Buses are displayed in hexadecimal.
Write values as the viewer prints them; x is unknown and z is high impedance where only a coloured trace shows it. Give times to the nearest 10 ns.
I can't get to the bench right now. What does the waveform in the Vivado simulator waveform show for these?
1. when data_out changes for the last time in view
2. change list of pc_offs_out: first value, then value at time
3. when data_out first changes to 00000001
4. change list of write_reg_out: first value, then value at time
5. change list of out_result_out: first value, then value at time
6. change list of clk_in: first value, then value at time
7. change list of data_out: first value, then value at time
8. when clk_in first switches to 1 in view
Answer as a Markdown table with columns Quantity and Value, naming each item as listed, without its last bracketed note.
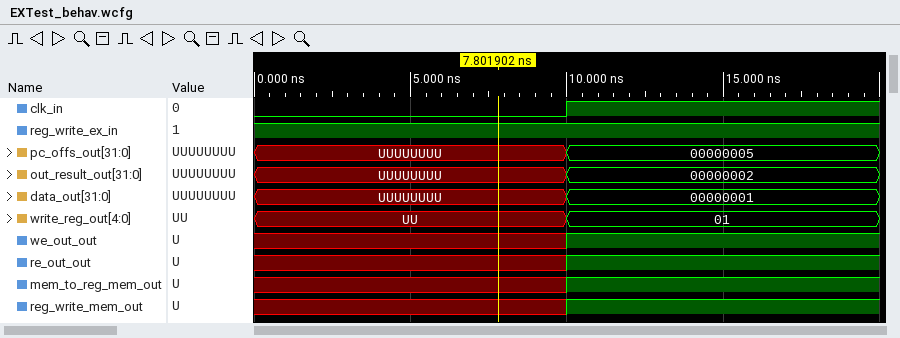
| Quantity | Value |
|---|---|
| when data_out changes for the last time in view | 10 ns |
| change list of pc_offs_out: first value, then value at time | UUUUUUUU, 00000005 at 10 ns |
| when data_out first changes to 00000001 | 10 ns |
| change list of write_reg_out: first value, then value at time | UU, 01 at 10 ns |
| change list of out_result_out: first value, then value at time | UUUUUUUU, 00000002 at 10 ns |
| change list of clk_in: first value, then value at time | 0, 1 at 10 ns |
| change list of data_out: first value, then value at time | UUUUUUUU, 00000001 at 10 ns |
| when clk_in first switches to 1 in view | 10 ns |
